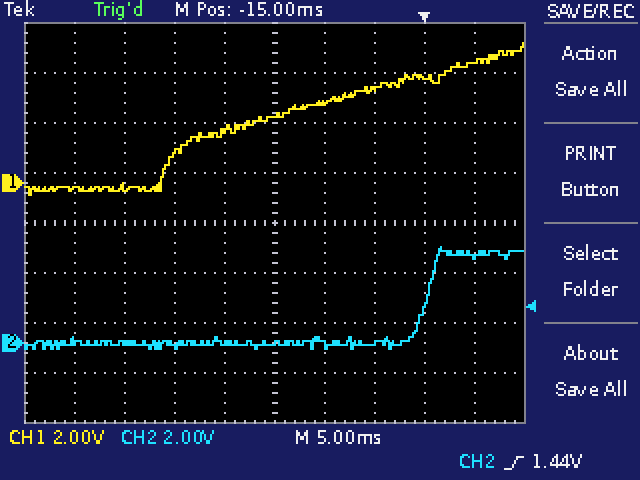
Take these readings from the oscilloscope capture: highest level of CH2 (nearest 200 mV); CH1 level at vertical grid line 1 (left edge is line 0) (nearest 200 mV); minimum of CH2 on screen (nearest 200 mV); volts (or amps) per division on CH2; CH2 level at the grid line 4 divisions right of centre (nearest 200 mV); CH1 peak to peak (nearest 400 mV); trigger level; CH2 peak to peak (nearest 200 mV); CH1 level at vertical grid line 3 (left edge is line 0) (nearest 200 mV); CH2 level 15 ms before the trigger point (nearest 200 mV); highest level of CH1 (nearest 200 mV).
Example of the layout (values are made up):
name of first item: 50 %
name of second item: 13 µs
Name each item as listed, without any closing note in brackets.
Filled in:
highest level of CH2: 3.8 V
CH1 level at vertical grid line 1 (left edge is line 0): -200 mV
minimum of CH2 on screen: -200 mV
volts (or amps) per division on CH2: 2 V
CH2 level at the grid line 4 divisions right of centre: 3.4 V
CH1 peak to peak: 6.0 V
trigger level: 1.44 V
CH2 peak to peak: 4.0 V
CH1 level at vertical grid line 3 (left edge is line 0): 1.2 V
CH2 level 15 ms before the trigger point: 0.0 V
highest level of CH1: 5.6 V
